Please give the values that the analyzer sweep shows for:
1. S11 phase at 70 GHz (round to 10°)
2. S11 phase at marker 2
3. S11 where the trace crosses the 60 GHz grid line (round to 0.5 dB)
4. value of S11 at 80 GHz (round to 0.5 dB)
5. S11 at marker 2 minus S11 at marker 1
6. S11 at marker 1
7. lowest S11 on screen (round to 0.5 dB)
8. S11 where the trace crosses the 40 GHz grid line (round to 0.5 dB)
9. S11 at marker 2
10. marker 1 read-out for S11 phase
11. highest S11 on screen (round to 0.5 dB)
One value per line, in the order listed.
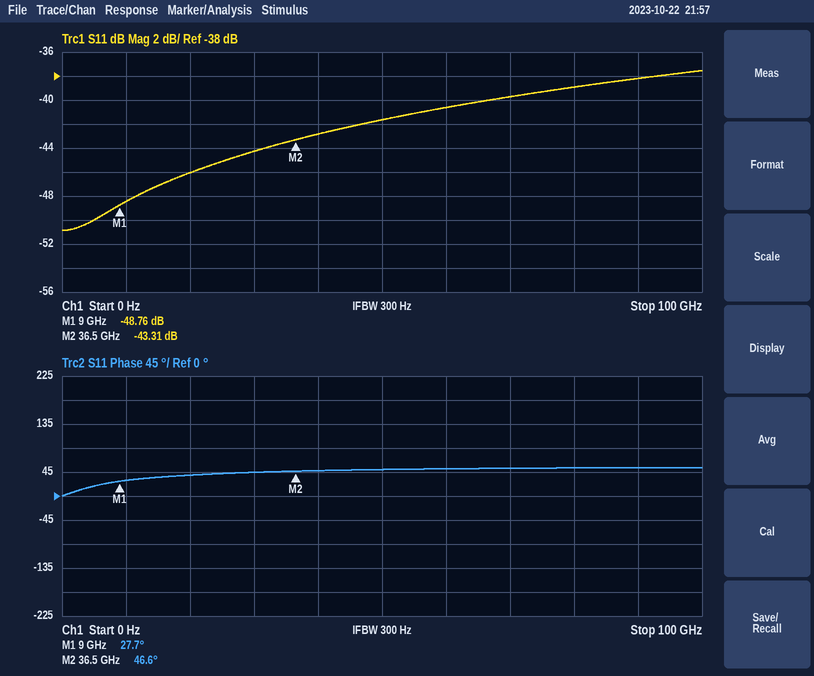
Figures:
50°
46.6°
-40.5 dB
-39.0 dB
5.45 dB
-48.76 dB
-51.0 dB
-43.0 dB
-43.31 dB
27.7°
-37.5 dB
